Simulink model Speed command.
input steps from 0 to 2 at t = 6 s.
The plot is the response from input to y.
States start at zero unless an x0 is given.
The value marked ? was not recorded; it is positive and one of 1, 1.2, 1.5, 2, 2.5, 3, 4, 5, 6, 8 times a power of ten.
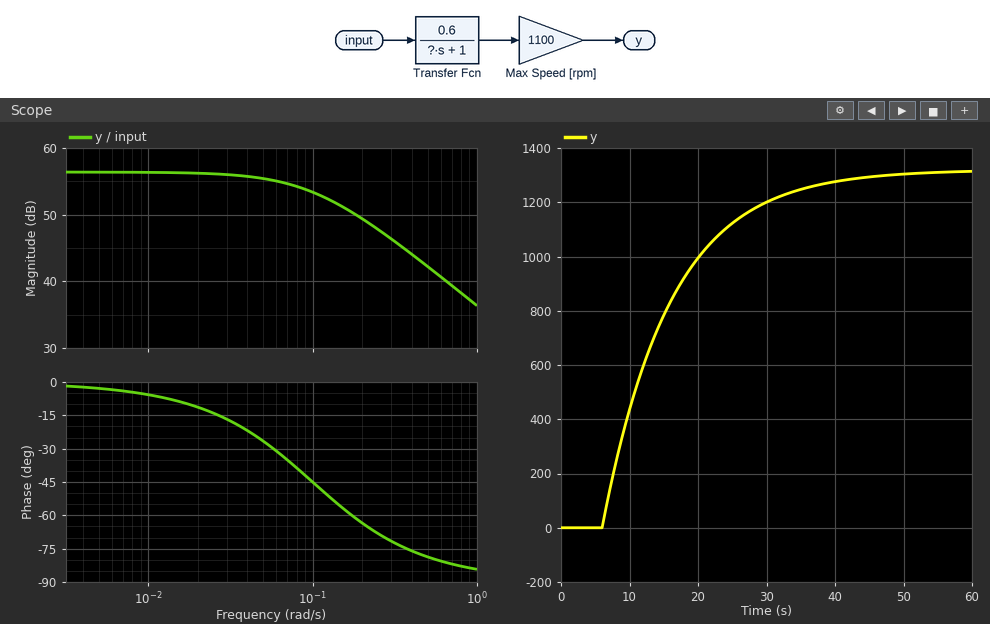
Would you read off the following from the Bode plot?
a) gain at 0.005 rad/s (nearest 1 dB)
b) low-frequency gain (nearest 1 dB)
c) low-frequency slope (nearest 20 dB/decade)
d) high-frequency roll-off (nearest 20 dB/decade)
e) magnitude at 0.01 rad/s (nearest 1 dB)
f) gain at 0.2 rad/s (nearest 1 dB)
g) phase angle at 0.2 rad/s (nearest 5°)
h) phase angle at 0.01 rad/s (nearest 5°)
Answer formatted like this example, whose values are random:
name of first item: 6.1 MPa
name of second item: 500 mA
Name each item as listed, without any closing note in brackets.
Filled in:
gain at 0.005 rad/s: 56 dB
low-frequency gain: 56 dB
low-frequency slope: 0 dB/decade
high-frequency roll-off: -20 dB/decade
magnitude at 0.01 rad/s: 56 dB
gain at 0.2 rad/s: 49 dB
phase angle at 0.2 rad/s: -65°
phase angle at 0.01 rad/s: -5°
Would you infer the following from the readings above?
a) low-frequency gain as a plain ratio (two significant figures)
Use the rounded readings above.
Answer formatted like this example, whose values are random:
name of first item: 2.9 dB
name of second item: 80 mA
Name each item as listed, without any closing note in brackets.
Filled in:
low-frequency gain as a plain ratio: 630
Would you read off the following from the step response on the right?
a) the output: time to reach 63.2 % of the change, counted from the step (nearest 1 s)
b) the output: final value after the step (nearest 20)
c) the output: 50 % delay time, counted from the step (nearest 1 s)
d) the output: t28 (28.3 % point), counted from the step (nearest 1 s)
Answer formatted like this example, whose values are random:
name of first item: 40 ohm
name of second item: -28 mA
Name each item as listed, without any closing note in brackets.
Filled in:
the output: time to reach 63.2 % of the change, counted from the step: 10 s
the output: final value after the step: 1320
the output: 50 % delay time, counted from the step: 7 s
the output: t28 (28.3 % point), counted from the step: 3 s
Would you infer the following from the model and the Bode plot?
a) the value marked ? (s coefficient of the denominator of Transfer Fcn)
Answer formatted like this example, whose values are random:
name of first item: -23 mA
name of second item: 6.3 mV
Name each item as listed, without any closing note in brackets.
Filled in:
the value marked ?: 10
